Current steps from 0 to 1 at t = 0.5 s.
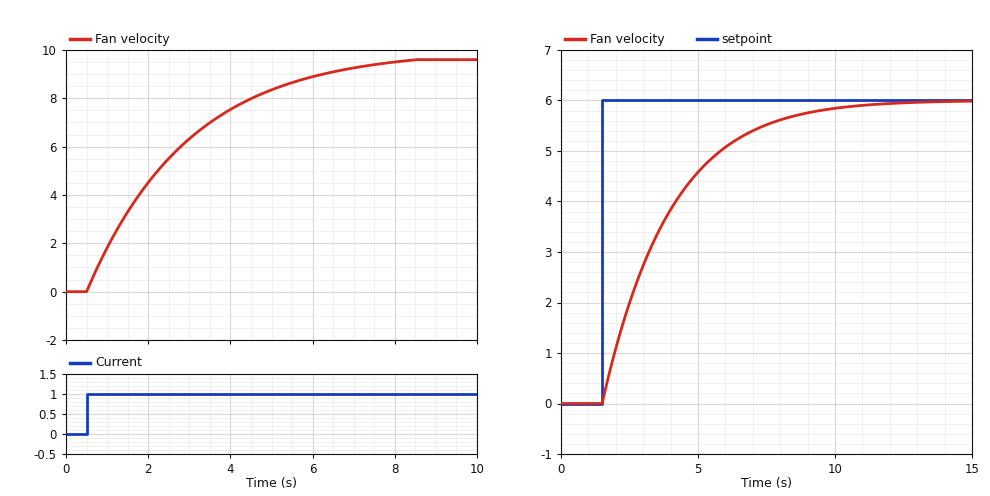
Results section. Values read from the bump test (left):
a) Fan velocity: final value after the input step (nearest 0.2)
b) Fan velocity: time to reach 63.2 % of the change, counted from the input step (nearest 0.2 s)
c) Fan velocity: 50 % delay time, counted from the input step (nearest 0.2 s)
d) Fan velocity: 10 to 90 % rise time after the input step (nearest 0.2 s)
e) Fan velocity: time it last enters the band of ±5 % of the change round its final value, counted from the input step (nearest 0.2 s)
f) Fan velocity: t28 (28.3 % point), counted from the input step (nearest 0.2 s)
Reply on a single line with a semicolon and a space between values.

9.6; 2.4 s; 1.6 s; 4.8 s; 6.0 s; 0.8 s
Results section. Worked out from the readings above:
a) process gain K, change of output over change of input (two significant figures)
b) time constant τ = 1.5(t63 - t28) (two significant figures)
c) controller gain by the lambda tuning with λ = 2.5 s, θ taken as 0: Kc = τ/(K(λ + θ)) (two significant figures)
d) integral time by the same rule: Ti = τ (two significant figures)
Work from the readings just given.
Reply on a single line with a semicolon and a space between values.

9.6; 2.4 s; 0.10; 2.4 s
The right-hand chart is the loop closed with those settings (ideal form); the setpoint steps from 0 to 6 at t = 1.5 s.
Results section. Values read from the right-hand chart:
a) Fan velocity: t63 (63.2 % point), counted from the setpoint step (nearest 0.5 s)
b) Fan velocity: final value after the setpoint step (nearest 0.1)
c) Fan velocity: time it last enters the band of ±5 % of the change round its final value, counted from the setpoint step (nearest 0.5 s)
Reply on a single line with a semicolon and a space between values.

2.5 s; 6.0; 7.0 s
